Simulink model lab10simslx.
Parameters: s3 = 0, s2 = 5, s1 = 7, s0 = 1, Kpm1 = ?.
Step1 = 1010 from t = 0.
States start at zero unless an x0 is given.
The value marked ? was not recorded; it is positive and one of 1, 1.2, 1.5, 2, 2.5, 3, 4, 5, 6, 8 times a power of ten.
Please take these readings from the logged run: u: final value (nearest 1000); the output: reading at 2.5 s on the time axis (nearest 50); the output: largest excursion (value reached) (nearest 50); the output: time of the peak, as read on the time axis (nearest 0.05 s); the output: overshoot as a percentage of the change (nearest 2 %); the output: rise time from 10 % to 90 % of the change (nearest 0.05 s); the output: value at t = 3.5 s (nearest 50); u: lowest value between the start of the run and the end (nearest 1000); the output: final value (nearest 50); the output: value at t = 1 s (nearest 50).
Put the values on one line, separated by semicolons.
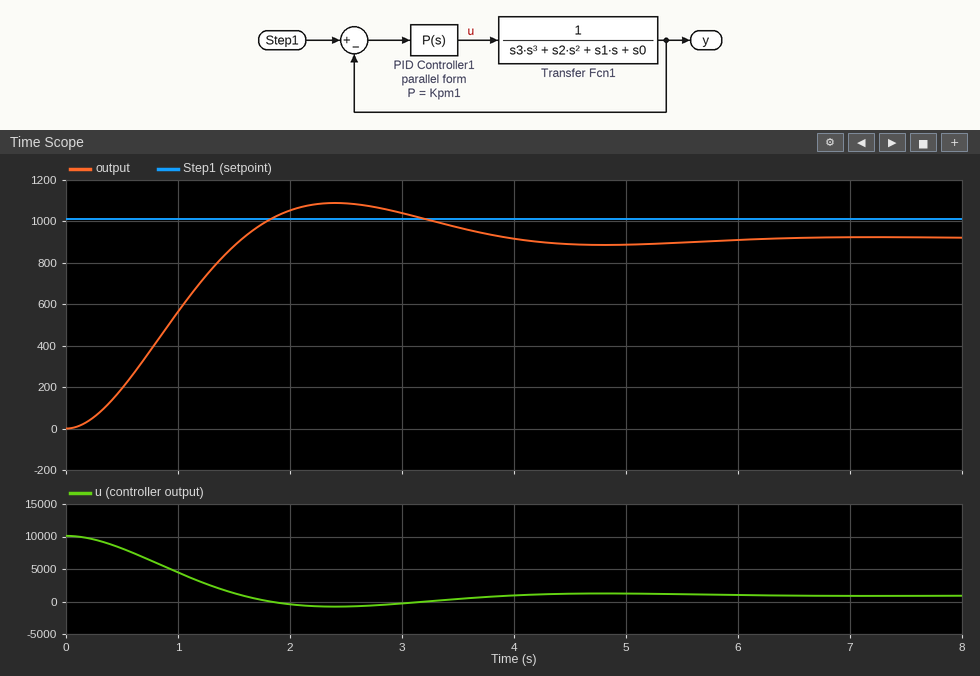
1000; 1100; 1100; 2.40 s; 18 %; 1.05 s; 950; -1000; 900; 550
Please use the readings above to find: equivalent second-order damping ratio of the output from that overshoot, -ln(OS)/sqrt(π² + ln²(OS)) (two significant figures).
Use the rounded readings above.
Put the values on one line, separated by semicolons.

0.48
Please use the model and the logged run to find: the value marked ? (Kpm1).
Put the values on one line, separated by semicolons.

10
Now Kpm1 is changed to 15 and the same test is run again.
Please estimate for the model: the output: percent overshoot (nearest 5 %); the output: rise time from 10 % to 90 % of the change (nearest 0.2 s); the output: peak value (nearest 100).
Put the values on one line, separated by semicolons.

25 %; 0.8 s; 1200
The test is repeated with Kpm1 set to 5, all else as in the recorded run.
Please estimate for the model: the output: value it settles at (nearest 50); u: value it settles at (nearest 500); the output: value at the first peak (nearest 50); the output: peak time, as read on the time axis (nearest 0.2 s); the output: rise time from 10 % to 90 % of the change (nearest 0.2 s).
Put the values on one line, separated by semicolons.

850; 1000; 900; 3.8 s; 1.8 s
